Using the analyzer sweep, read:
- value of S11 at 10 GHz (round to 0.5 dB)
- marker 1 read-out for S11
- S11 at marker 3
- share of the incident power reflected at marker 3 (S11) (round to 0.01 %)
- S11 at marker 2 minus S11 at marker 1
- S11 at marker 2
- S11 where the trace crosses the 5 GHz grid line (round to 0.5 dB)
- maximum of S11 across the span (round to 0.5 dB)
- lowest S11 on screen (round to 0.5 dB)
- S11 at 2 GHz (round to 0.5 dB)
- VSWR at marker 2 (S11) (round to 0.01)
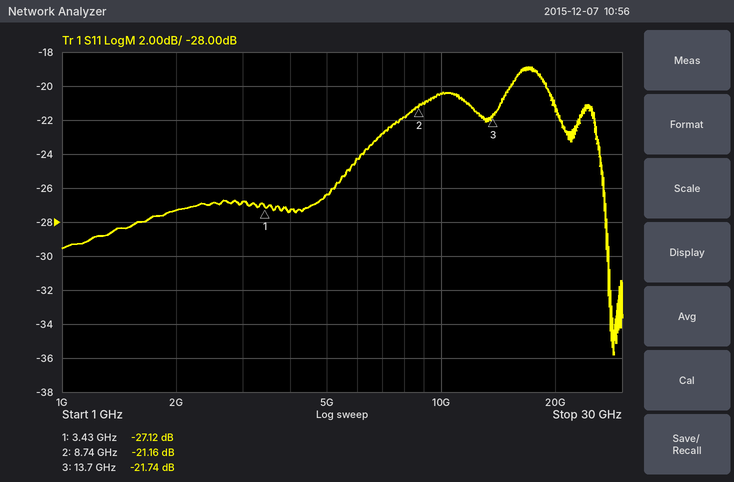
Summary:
-20.5 dB
-27.12 dB
-21.74 dB
0.67 %
5.96 dB
-21.16 dB
-26.5 dB
-19.0 dB
-36.0 dB
-27.5 dB
1.19
